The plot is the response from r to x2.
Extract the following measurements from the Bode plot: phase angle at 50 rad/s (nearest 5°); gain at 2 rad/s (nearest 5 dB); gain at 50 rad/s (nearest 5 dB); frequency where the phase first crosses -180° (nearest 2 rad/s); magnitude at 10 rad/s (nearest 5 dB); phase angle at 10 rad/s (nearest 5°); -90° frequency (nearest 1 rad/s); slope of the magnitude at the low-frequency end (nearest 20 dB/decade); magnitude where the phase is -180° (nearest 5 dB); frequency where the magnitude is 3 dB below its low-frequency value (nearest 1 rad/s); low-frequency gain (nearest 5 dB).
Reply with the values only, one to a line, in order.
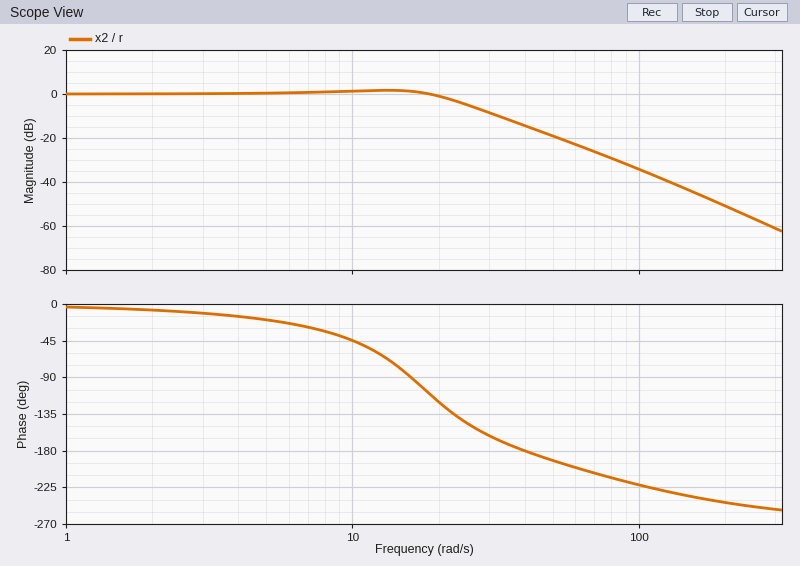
-190°
0 dB
-20 dB
40 rad/s
0 dB
-45°
16 rad/s
0 dB/decade
-15 dB
23 rad/s
0 dB
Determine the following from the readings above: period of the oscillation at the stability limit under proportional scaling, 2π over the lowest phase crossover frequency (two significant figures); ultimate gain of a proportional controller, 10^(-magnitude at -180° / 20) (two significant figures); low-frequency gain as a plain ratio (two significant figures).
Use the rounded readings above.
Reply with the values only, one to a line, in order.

0.16 s
5.6
1.0
